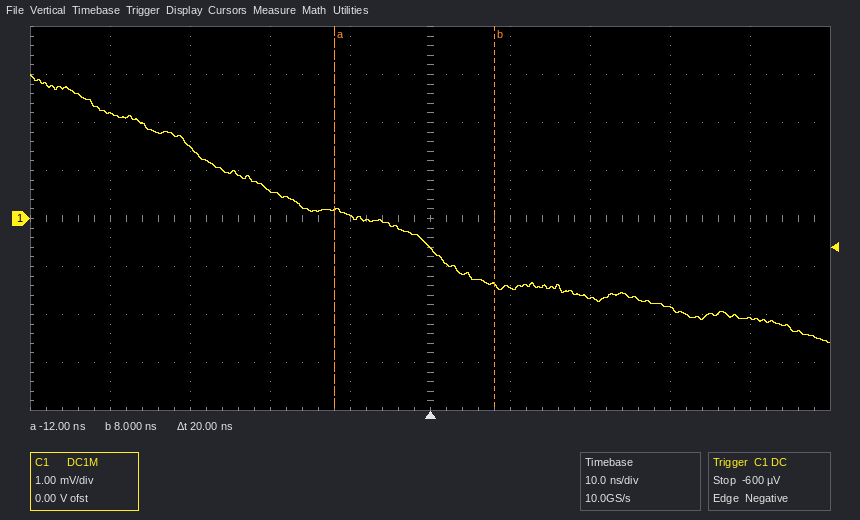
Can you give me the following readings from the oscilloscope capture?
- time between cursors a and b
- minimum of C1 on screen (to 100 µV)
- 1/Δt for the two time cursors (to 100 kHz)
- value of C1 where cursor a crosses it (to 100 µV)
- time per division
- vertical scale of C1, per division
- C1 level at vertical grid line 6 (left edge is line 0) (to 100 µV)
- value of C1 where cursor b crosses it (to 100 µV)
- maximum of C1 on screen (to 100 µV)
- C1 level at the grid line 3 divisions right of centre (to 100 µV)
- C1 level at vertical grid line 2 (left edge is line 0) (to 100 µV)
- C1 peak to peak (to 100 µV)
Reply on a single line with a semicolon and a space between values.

20 ns; -2.6 mV; 50.0 MHz; 200 µV; 10 ns; 1 mV; -1.4 mV; -1.4 mV; 3.0 mV; -1.9 mV; 1.5 mV; 5.6 mV
